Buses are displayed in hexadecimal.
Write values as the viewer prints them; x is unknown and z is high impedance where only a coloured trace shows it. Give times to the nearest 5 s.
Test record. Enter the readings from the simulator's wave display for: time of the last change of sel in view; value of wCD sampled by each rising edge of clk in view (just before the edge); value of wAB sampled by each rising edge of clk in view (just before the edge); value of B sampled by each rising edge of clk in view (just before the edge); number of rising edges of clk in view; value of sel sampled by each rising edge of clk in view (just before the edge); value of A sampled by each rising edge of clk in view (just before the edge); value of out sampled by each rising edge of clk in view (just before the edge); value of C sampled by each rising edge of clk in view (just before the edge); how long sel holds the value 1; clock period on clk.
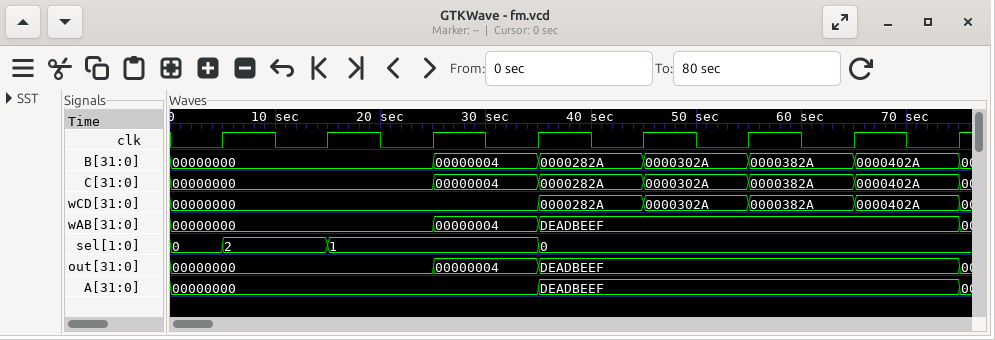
35 s
00000000, 00000000, 00000000, 00000000, 0000282A, 0000302A, 0000382A, 0000402A
00000000, 00000000, 00000000, 00000004, DEADBEEF, DEADBEEF, DEADBEEF, DEADBEEF
00000000, 00000000, 00000000, 00000004, 0000282A, 0000302A, 0000382A, 0000402A
8
0, 2, 1, 1, 0, 0, 0, 0
00000000, 00000000, 00000000, 00000000, DEADBEEF, DEADBEEF, DEADBEEF, DEADBEEF
00000000, 00000000, 00000000, 00000004, DEADBEEF, DEADBEEF, DEADBEEF, DEADBEEF
00000000, 00000000, 00000000, 00000004, 0000282A, 0000302A, 0000382A, 0000402A
20 s
10 s
